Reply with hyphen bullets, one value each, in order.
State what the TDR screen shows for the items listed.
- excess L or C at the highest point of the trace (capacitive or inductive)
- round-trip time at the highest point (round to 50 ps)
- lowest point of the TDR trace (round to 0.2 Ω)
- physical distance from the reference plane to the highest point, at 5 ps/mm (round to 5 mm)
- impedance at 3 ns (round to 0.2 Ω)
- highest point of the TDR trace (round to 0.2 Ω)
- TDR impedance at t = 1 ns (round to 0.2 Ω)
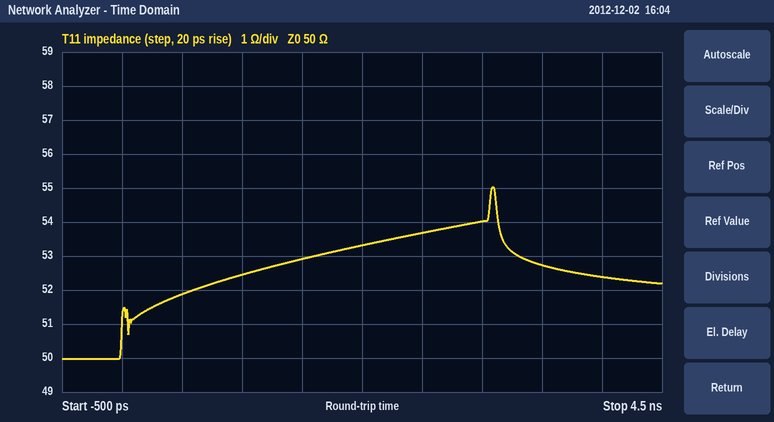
- inductive
- 3.10 ns
- 50.0 Ω
- 310 mm
- 54.0 Ω
- 55.0 Ω
- 52.4 Ω
